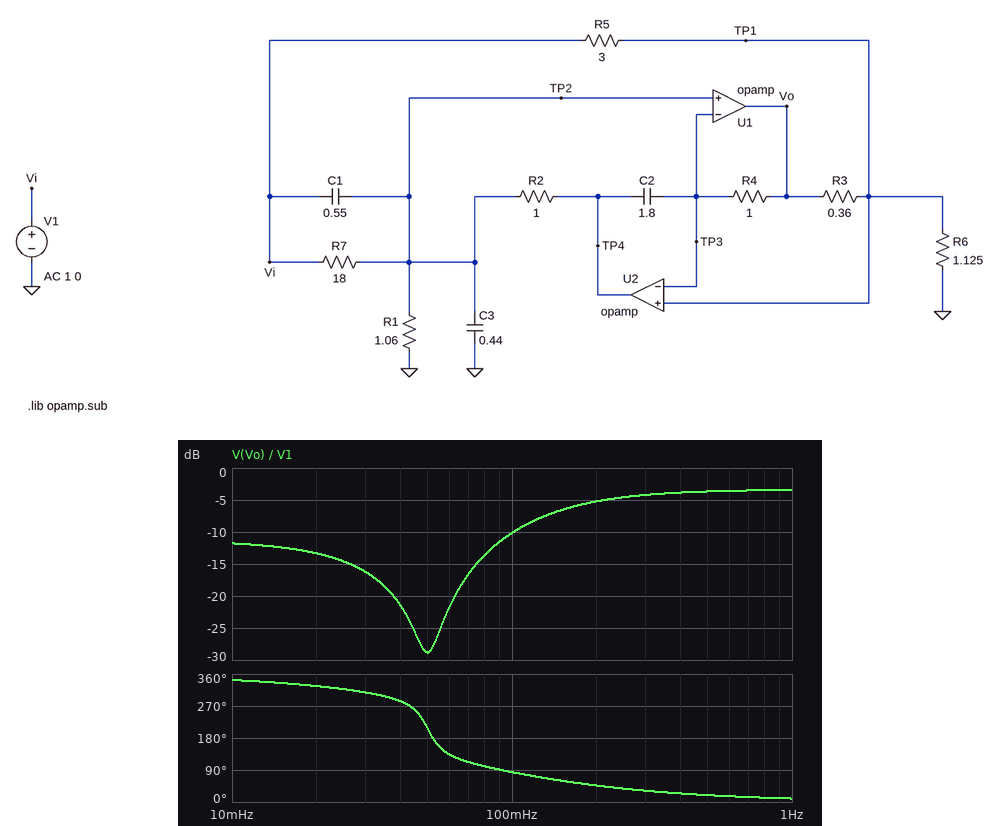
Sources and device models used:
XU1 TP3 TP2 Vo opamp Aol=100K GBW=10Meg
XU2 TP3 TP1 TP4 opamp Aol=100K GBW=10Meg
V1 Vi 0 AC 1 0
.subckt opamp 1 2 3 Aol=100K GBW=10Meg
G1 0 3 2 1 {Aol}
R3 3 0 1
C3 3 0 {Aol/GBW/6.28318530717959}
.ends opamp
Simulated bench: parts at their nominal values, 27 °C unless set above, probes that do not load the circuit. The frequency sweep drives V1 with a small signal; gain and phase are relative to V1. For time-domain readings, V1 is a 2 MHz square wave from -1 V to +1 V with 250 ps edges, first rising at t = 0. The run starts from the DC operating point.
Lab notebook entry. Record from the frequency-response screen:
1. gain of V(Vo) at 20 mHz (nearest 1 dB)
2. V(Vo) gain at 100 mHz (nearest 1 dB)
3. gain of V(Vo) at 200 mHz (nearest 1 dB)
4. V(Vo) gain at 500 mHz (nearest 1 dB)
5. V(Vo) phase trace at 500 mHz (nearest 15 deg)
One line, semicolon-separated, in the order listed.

-13 dB; -10 dB; -5 dB; -4 dB; 15 deg
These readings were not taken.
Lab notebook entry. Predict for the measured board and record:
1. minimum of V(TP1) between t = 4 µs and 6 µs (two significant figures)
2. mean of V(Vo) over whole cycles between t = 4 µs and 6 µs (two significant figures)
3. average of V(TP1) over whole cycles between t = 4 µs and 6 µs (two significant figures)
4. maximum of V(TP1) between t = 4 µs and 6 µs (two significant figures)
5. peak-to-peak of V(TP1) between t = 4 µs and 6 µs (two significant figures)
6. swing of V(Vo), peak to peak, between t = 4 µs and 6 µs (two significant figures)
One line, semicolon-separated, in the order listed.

-450 mV; 410 mV; 280 mV; 1.0 V; 1.5 V; 1.9 V
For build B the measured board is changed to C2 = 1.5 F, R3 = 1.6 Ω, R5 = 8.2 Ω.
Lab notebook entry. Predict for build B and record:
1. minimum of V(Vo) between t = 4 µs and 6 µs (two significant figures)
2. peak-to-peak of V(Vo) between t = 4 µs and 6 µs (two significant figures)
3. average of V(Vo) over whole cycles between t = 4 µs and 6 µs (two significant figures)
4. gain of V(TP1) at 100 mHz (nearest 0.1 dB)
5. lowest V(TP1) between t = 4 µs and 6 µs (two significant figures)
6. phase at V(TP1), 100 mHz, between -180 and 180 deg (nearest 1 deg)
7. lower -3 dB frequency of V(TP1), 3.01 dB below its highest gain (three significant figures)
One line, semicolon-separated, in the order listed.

-180 mV; 2.6 V; 1.1 V; -19.9 dB; -140 mV; 116 deg; 159 mHz
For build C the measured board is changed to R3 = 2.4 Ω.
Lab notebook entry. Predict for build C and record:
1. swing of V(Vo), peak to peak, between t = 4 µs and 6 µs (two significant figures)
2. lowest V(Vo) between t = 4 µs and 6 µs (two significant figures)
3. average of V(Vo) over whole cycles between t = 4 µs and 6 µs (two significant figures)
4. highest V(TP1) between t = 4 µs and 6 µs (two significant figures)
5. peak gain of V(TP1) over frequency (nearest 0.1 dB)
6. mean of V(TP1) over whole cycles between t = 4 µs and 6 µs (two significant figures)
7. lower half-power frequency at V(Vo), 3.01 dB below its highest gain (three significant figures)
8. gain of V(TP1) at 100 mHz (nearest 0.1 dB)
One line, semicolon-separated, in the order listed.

2.8 V; -270 mV; 1.1 V; 840 mV; -4.8 dB; 280 mV; 180 mHz; -15.6 dB
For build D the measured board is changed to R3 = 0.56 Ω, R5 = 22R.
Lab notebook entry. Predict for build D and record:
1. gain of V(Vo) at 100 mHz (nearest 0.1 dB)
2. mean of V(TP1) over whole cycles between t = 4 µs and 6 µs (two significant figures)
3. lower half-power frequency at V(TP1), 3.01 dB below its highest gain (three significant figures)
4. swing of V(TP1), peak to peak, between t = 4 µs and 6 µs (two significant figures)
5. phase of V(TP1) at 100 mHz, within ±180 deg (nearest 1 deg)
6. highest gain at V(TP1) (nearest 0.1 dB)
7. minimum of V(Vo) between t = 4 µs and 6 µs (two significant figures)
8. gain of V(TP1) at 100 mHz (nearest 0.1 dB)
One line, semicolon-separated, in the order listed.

-6.3 dB; 510 mV; 128 mHz; 1.4 V; 71 deg; -5.1 dB; -290 mV; -9.8 dB
